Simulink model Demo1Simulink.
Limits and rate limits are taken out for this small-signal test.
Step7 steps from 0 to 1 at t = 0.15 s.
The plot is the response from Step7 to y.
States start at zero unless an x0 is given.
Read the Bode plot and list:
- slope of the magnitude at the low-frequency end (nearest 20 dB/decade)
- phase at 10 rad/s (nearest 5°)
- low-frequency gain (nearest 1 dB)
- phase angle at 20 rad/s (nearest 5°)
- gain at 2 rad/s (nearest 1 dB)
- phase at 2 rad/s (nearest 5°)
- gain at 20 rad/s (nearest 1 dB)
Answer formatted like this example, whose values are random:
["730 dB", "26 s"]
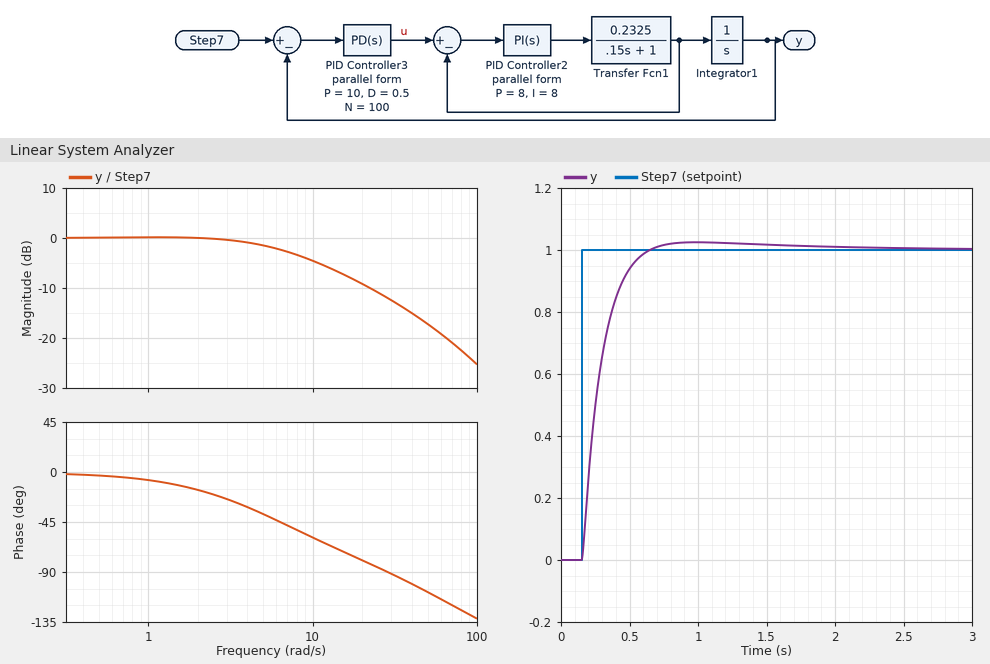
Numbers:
["0 dB/decade", "-60°", "0 dB", "-80°", "0 dB", "-15°", "-9 dB"]
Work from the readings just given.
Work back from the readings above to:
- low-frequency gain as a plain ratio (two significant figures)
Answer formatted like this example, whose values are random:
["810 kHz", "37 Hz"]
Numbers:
["1.0"]
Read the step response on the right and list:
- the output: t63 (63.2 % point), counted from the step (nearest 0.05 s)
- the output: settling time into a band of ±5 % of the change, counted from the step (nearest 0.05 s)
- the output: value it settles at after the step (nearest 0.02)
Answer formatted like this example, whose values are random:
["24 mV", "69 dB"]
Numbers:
["0.15 s", "0.35 s", "1.00"]
